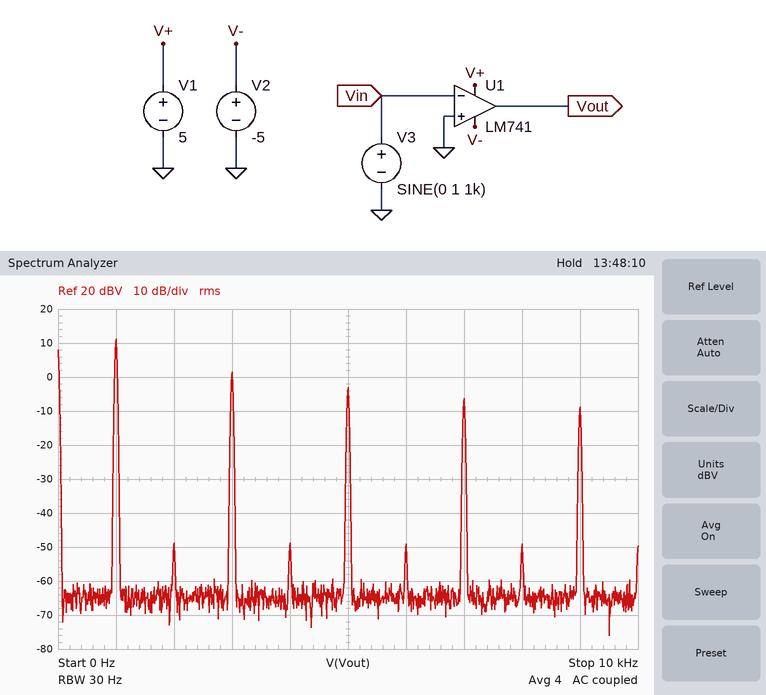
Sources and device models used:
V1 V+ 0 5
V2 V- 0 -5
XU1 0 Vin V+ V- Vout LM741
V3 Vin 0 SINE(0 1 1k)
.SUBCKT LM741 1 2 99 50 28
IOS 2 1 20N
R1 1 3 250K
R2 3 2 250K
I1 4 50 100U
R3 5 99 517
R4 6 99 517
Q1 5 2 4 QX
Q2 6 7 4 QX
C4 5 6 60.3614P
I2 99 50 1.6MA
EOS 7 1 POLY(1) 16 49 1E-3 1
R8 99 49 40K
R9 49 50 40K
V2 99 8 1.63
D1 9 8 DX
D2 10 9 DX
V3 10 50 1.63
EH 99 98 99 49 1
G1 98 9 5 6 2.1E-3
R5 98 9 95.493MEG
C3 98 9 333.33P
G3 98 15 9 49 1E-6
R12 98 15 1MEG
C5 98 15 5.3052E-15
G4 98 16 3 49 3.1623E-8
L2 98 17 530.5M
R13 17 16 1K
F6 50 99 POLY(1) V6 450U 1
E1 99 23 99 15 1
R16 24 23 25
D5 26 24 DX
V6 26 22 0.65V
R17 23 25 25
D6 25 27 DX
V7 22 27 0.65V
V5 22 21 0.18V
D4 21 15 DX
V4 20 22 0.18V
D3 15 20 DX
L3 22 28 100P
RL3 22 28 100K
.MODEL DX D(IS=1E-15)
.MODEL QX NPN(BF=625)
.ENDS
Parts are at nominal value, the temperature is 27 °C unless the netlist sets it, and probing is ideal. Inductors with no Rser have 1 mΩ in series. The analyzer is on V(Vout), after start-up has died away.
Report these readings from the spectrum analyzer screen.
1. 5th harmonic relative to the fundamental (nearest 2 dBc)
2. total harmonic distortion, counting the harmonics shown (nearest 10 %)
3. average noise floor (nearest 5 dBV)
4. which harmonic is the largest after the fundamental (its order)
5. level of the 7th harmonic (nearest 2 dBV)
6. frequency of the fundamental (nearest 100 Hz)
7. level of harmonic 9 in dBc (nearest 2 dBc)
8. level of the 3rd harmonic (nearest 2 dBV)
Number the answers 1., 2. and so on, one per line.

1. -14 dBc
2. 40 %
3. -65 dBV
4. 3
5. -6 dBV
6. 1.0 kHz
7. -20 dBc
8. 2 dBV
